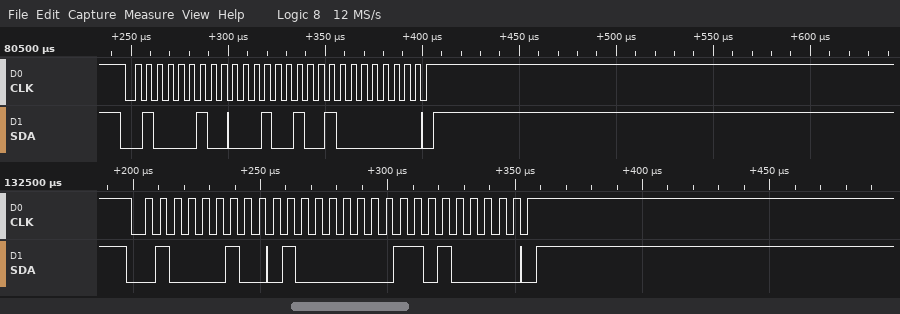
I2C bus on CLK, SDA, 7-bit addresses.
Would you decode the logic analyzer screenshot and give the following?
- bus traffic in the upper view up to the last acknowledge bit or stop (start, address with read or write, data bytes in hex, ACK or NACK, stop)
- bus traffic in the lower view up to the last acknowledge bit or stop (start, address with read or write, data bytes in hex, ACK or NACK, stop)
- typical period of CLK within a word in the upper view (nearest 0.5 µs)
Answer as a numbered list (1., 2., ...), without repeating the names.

1. start, address 21 write ACK, 12 ACK, 80 ACK, stop
2. start, address 21 write ACK, 40 ACK, D0 ACK, stop
3. 5.5 µs
